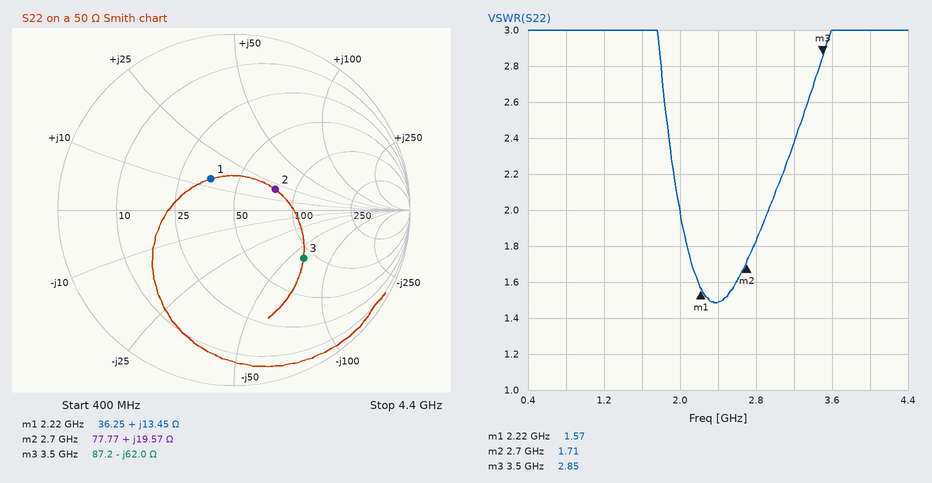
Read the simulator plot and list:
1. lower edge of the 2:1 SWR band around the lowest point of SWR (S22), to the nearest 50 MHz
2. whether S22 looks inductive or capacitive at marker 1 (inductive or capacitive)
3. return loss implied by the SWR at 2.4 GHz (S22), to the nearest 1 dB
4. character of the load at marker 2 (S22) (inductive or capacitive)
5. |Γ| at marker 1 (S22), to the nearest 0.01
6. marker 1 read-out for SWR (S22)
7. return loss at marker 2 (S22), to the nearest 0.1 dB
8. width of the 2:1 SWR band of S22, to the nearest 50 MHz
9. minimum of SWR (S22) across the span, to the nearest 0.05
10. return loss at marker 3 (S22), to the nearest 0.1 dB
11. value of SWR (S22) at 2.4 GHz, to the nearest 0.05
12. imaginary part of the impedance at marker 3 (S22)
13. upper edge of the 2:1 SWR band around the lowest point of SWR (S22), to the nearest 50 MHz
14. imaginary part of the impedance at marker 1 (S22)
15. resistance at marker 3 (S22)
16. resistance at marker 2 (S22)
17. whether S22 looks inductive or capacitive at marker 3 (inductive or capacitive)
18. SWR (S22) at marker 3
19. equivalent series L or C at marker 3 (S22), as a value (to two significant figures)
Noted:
2.00 GHz
inductive
14 dB
inductive
0.22
1.57
11.6 dB
950 MHz
1.50
6.4 dB
1.50
-62.0 Ω
2.95 GHz
+13.45 Ω
87.2 Ω
77.77 Ω
capacitive
2.85
730 fF
